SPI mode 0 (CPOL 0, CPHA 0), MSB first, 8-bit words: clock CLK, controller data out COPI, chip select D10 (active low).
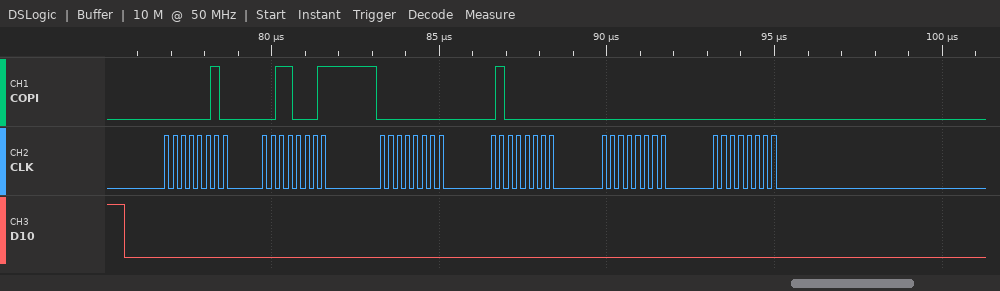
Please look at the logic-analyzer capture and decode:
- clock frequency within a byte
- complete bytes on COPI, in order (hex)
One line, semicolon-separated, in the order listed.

4 MHz; 0x02 0x31 0x00 0x40 0x00 0x00
